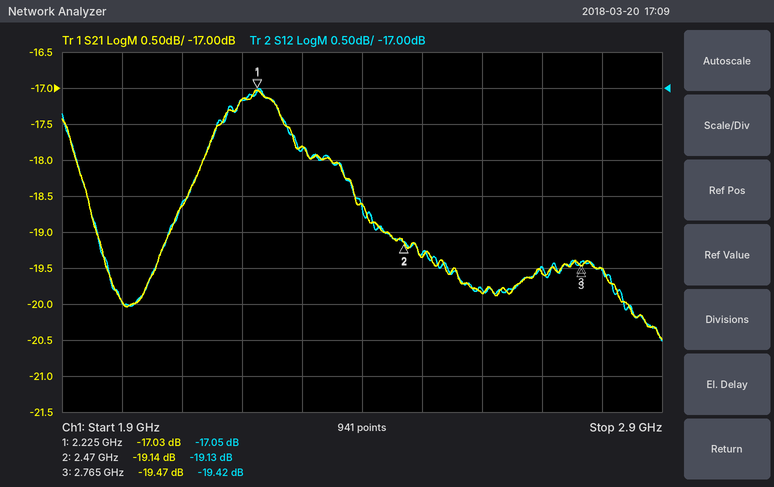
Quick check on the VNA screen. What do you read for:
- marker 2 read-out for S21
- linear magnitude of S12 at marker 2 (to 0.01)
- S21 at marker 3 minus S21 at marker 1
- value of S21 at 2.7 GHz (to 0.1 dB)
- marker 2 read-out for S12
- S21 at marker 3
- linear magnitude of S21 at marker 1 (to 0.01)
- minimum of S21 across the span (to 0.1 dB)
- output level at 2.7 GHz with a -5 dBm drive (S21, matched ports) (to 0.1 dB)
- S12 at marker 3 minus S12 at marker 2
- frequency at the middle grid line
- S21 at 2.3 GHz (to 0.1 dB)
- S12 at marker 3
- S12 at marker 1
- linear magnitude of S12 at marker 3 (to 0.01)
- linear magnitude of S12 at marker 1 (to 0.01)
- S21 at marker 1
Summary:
-19.14 dB
0.11
-2.44 dB
-19.6 dB
-19.13 dB
-19.47 dB
0.14
-20.5 dB
-24.6 dBm
-0.29 dB
2.4 GHz
-17.8 dB
-19.42 dB
-17.05 dB
0.11
0.14
-17.03 dB
